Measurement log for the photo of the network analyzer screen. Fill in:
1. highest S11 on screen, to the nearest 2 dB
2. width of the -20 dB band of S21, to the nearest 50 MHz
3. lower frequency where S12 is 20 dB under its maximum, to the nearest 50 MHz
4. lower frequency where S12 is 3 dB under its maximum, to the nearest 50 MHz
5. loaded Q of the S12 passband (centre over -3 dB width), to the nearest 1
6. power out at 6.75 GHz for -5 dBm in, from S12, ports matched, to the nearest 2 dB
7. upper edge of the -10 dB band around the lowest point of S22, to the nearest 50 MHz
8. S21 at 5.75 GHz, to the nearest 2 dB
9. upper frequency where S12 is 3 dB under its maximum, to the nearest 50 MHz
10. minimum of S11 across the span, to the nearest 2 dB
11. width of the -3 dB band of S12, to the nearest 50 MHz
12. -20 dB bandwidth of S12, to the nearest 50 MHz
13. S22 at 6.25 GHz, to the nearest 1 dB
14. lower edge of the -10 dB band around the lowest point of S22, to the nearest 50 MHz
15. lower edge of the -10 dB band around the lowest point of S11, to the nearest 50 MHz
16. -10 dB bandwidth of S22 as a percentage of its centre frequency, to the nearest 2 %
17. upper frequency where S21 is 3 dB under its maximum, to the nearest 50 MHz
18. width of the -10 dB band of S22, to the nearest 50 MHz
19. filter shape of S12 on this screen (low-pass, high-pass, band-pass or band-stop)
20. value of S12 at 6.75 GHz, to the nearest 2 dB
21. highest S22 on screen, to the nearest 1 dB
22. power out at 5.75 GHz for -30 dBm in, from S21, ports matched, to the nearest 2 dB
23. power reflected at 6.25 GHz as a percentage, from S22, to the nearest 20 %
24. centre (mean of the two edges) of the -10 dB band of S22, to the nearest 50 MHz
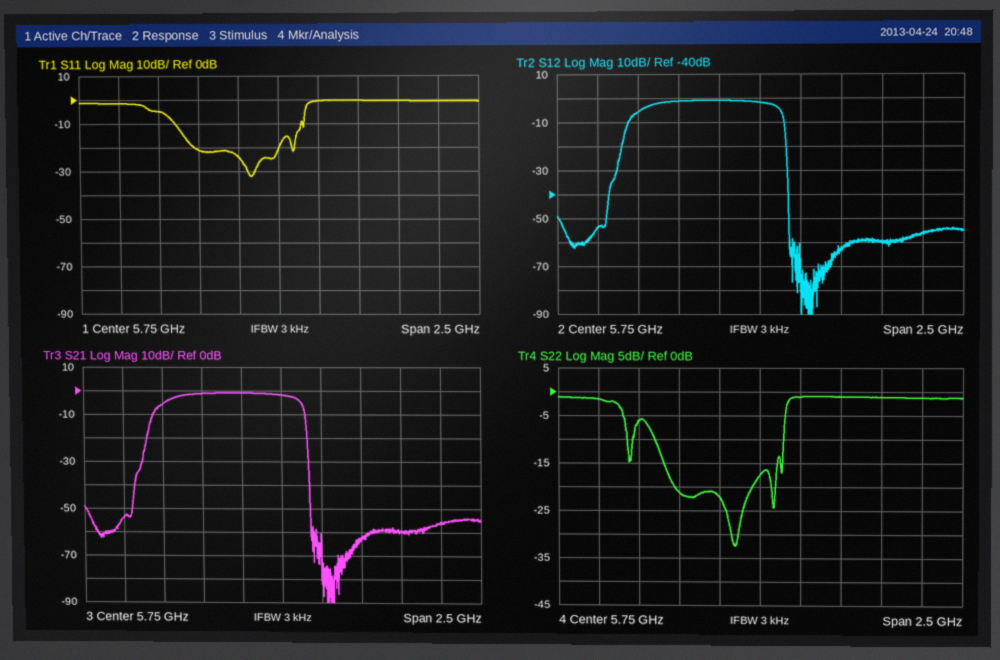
0 dB
1.00 GHz
4.90 GHz
5.05 GHz
7
-62 dBm
5.90 GHz
-2 dB
5.85 GHz
-32 dB
800 MHz
1.00 GHz
-1 dB
5.10 GHz
5.10 GHz
14 %
5.85 GHz
800 MHz
band-pass
-56 dB
-1 dB
-32 dBm
80 %
5.50 GHz
